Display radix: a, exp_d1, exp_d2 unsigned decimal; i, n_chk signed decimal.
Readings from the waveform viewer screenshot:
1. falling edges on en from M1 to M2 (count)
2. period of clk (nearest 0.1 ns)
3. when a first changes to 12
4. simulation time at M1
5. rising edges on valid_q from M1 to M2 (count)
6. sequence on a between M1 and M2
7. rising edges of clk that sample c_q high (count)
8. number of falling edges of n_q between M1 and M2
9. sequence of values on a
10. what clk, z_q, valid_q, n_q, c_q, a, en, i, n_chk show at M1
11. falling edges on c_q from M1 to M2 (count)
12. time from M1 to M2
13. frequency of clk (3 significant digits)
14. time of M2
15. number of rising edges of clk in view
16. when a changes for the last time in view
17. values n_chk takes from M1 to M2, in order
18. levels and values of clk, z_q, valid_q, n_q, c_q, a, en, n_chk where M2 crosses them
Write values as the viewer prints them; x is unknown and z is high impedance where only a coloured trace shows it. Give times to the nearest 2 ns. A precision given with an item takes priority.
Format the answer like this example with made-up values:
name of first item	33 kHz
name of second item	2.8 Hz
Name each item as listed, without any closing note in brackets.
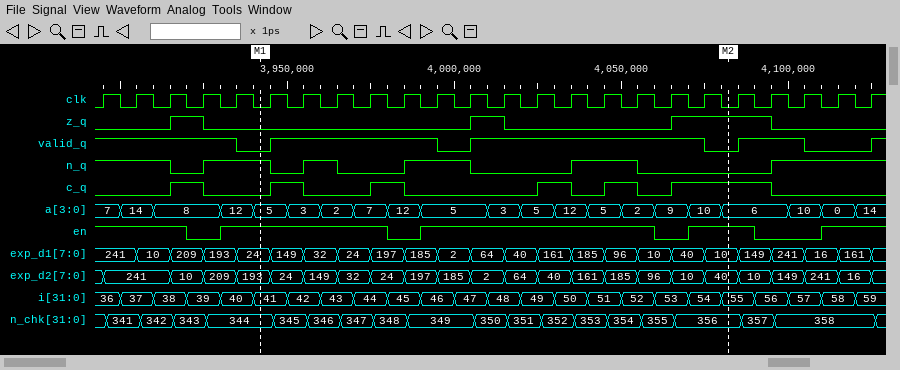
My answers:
falling edges on en from M1 to M2	2
period of clk	10 ns
when a first changes to 12	3930 ns
simulation time at M1	3942 ns
rising edges on valid_q from M1 to M2	2
sequence on a between M1 and M2	5, 3, 2, 7, 12, 5, 3, 5, 12, 5, 2, 9, 10, 6
rising edges of clk that sample c_q high	8
number of falling edges of n_q between M1 and M2	4
sequence of values on a	7, 14, 8, 12, 5, 3, 2, 7, 12, 5, 3, 5, 12, 5, 2, 9, 10, 6, 10, 0, 14
what clk, z_q, valid_q, n_q, c_q, a, en, i, n_chk show at M1	clk=0, z_q=0, valid_q=0, n_q=1, c_q=0, a=5, en=1, i=41, n_chk=344
falling edges on c_q from M1 to M2	4
time from M1 to M2	140 ns
frequency of clk	100 MHz
time of M2	4082 ns
number of rising edges of clk in view	24
when a changes for the last time in view	4120 ns
values n_chk takes from M1 to M2, in order	344, 345, 346, 347, 348, 349, 350, 351, 352, 353, 354, 355, 356
levels and values of clk, z_q, valid_q, n_q, c_q, a, en, n_chk where M2 crosses them	clk=0, z_q=1, valid_q=0, n_q=0, c_q=1, a=6, en=1, n_chk=356
